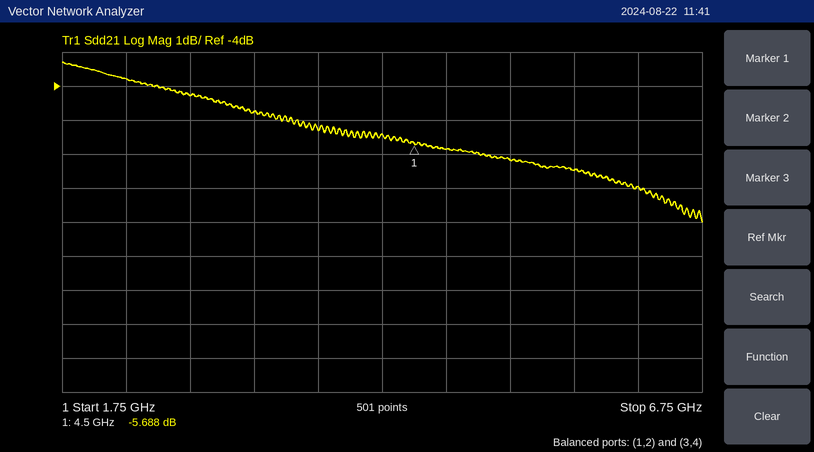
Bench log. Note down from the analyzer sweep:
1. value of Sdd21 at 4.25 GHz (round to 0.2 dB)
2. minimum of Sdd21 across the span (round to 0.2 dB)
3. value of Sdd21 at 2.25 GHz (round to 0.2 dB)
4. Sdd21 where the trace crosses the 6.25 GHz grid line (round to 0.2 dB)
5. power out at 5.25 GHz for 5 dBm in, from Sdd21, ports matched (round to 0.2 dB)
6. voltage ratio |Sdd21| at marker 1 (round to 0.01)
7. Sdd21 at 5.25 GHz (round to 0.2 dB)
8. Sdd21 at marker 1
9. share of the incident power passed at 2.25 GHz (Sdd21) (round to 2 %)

-5.4 dB
-8.0 dB
-3.8 dB
-7.0 dB
-1.2 dBm
0.52
-6.2 dB
-5.688 dB
42 %
